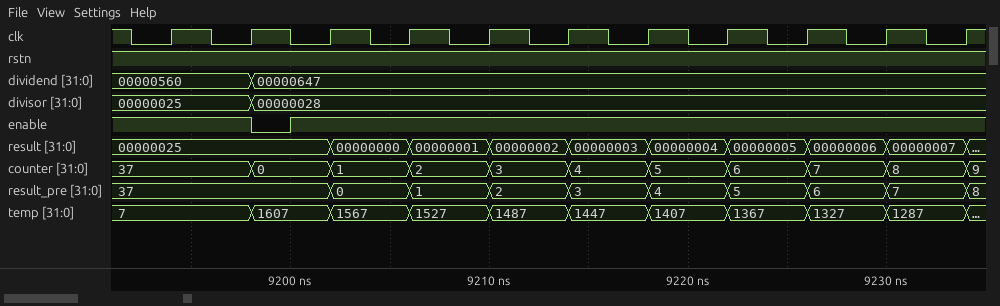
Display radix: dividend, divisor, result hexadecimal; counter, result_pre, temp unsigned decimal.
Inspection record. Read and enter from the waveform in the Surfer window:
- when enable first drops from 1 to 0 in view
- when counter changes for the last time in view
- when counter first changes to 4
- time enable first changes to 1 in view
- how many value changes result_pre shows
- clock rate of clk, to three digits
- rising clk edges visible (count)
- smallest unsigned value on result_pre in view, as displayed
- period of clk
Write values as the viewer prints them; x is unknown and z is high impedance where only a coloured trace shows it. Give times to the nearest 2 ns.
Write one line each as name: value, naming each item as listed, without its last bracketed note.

when enable first drops from 1 to 0 in view: 9198 ns
when counter changes for the last time in view: 9234 ns
when counter first changes to 4: 9214 ns
time enable first changes to 1 in view: 9200 ns
how many value changes result_pre shows: 9
clock rate of clk, to three digits: 250 MHz
rising clk edges visible: 11
smallest unsigned value on result_pre in view, as displayed: 0
period of clk: 4 ns
